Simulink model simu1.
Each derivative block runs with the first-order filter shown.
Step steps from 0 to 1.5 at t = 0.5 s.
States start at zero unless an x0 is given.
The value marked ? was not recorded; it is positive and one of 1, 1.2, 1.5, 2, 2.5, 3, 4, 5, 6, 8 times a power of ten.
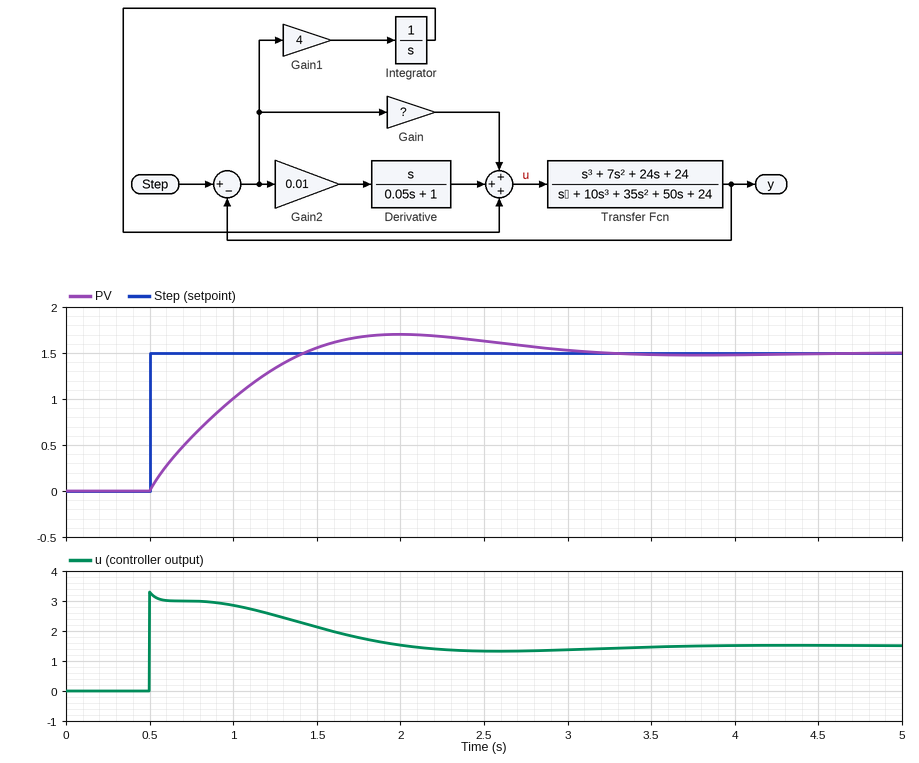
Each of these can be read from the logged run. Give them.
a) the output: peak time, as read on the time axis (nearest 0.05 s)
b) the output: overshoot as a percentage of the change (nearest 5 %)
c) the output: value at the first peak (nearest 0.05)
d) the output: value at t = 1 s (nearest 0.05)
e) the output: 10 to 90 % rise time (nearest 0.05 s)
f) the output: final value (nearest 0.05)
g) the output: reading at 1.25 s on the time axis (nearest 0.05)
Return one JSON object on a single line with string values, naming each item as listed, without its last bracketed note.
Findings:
{"the output: peak time, as read on the time axis": "2.00 s", "the output: overshoot as a percentage of the change": "15 %", "the output: value at the first peak": "1.70", "the output: value at t = 1 s": "1.00", "the output: 10 to 90 % rise time": "0.70 s", "the output: final value": "1.50", "the output: reading at 1.25 s on the time axis": "1.35"}
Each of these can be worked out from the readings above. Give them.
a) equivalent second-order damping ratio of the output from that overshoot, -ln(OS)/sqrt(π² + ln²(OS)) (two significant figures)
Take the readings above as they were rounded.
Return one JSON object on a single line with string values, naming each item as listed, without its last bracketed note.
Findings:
{"equivalent second-order damping ratio of the output from that overshoot, -ln(OS)/sqrt(π² + ln²(OS))": "0.52"}
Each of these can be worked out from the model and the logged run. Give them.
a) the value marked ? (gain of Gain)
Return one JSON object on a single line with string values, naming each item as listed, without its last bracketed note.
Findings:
{"the value marked ?": "2"}
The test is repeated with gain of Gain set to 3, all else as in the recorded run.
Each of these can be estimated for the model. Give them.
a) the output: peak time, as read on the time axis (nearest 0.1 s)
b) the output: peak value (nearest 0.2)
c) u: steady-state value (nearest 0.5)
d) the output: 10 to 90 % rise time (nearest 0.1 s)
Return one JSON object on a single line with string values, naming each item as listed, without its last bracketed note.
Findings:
{"the output: peak time, as read on the time axis": "1.9 s", "the output: peak value": "1.6", "u: steady-state value": "1.5", "the output: 10 to 90 % rise time": "0.7 s"}
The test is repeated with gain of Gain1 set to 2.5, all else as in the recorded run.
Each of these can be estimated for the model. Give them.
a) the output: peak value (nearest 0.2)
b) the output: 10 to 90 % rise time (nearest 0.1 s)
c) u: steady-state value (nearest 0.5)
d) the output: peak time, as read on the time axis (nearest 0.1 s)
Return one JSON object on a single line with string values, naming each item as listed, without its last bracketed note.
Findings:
{"the output: peak value": "1.6", "the output: 10 to 90 % rise time": "0.9 s", "u: steady-state value": "1.5", "the output: peak time, as read on the time axis": "2.3 s"}
